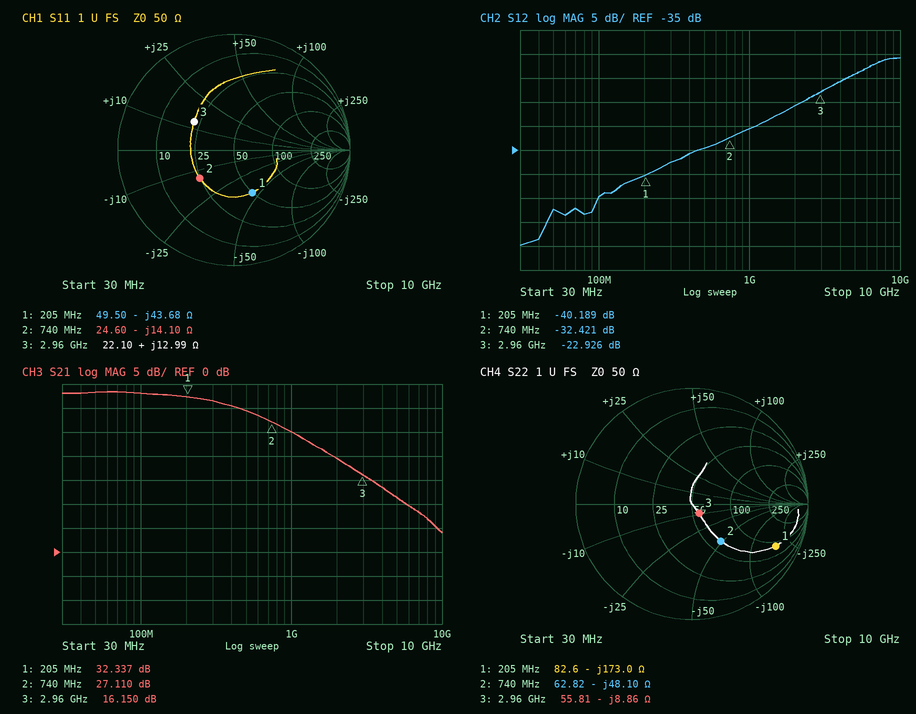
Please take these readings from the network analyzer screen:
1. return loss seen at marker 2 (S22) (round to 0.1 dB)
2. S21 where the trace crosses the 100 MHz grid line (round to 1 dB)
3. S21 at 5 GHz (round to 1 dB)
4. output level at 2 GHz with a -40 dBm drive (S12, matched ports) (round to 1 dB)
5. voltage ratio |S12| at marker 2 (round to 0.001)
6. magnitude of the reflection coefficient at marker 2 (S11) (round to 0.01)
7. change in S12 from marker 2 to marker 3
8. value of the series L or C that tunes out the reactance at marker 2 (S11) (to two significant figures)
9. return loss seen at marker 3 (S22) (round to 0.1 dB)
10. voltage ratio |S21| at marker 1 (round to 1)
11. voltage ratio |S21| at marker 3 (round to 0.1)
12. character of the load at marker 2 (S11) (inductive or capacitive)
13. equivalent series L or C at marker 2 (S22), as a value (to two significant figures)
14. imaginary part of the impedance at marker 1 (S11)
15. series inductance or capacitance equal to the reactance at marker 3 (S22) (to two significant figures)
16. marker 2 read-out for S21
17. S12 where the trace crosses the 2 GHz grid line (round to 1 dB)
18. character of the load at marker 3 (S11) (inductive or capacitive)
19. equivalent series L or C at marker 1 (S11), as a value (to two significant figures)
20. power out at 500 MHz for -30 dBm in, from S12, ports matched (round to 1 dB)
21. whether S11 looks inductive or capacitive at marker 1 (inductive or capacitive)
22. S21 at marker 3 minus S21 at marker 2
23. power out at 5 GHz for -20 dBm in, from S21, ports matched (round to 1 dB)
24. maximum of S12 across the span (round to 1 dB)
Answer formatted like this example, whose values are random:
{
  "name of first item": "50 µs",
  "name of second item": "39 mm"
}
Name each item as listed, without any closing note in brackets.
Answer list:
{
  "return loss seen at marker 2 (S22)": "7.8 dB",
  "S21 where the trace crosses the 100 MHz grid line": "33 dB",
  "S21 at 5 GHz": "11 dB",
  "output level at 2 GHz with a -40 dBm drive (S12, matched ports)": "-66 dBm",
  "voltage ratio |S12| at marker 2": "0.024",
  "magnitude of the reflection coefficient at marker 2 (S11)": "0.38",
  "change in S12 from marker 2 to marker 3": "9.495 dB",
  "value of the series L or C that tunes out the reactance at marker 2 (S11)": "3.0 nH",
  "return loss seen at marker 3 (S22)": "20.0 dB",
  "voltage ratio |S21| at marker 1": "41",
  "voltage ratio |S21| at marker 3": "6.4",
  "character of the load at marker 2 (S11)": "capacitive",
  "equivalent series L or C at marker 2 (S22), as a value": "4.5 pF",
  "imaginary part of the impedance at marker 1": "-43.68 Ω",
  "series inductance or capacitance equal to the reactance at marker 3 (S22)": "6.1 pF",
  "marker 2 read-out for S21": "27.110 dB",
  "S12 where the trace crosses the 2 GHz grid line": "-26 dB",
  "character of the load at marker 3 (S11)": "inductive",
  "equivalent series L or C at marker 1 (S11), as a value": "18 pF",
  "power out at 500 MHz for -30 dBm in, from S12, ports matched": "-65 dBm",
  "whether S11 looks inductive or capacitive at marker 1": "capacitive",
  "S21 at marker 3 minus S21 at marker 2": "-10.960 dB",
  "power out at 5 GHz for -20 dBm in, from S21, ports matched": "-9 dBm",
  "maximum of S12 across the span": "-16 dB"
}
